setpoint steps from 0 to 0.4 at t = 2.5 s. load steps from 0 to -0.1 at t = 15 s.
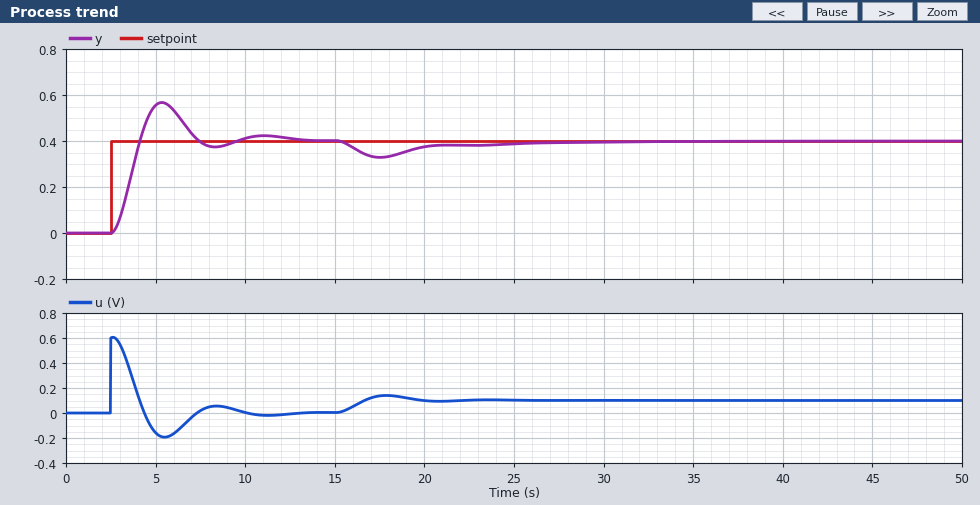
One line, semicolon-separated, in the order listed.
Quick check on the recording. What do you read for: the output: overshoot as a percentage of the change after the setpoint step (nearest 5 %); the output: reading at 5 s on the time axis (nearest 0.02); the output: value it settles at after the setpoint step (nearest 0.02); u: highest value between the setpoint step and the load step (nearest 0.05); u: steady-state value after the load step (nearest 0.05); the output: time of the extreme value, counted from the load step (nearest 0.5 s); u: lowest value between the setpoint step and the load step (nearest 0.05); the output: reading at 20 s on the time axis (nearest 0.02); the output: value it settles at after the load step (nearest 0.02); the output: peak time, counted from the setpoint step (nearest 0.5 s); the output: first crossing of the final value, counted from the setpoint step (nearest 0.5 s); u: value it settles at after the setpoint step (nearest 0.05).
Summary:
40 %; 0.56; 0.40; 0.60; 0.10; 2.5 s; -0.20; 0.38; 0.40; 3.0 s; 1.5 s; 0.00
